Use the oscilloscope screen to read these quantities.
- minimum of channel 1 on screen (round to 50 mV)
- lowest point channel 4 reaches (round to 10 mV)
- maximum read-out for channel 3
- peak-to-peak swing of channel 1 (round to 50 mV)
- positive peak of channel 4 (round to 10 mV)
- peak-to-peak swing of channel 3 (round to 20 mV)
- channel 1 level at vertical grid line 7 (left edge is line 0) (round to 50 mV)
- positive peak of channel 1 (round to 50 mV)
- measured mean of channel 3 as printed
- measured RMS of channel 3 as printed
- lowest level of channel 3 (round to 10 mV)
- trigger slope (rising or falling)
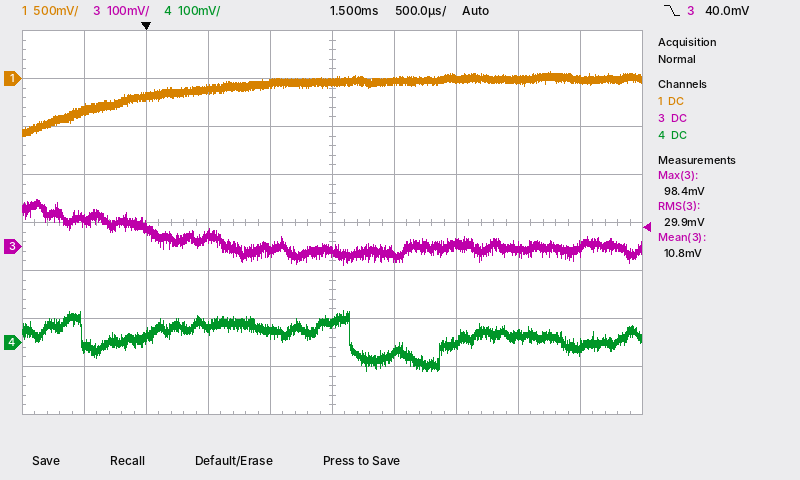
-600 mV
-60 mV
98.4 mV
650 mV
70 mV
140 mV
0 mV
50 mV
10.8 mV
29.9 mV
-40 mV
falling
